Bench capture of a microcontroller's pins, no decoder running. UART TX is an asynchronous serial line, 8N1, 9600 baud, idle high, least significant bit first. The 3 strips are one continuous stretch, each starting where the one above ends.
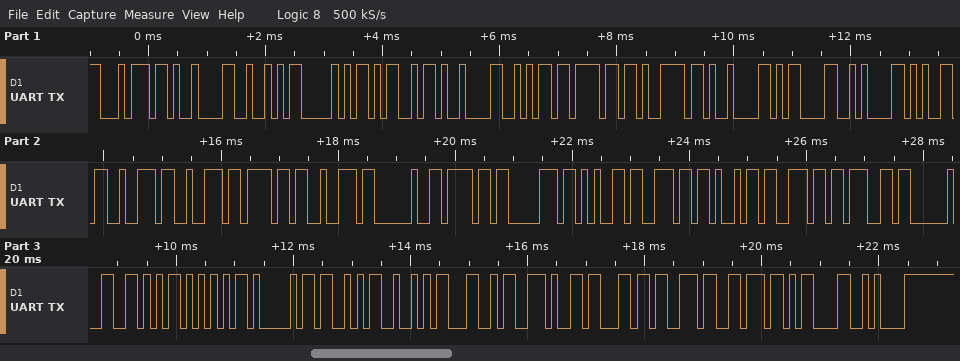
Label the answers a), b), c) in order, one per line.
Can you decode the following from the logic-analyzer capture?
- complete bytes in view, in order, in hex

a) 74 09 52 50 4D 09 6A 6F 79 09 0D 0A 65 72 72 6F 72 20 6F 70 65 6E 69 6E 67 20 56 55 41 53 52 4C 2E 63 73 76 0D 0A
